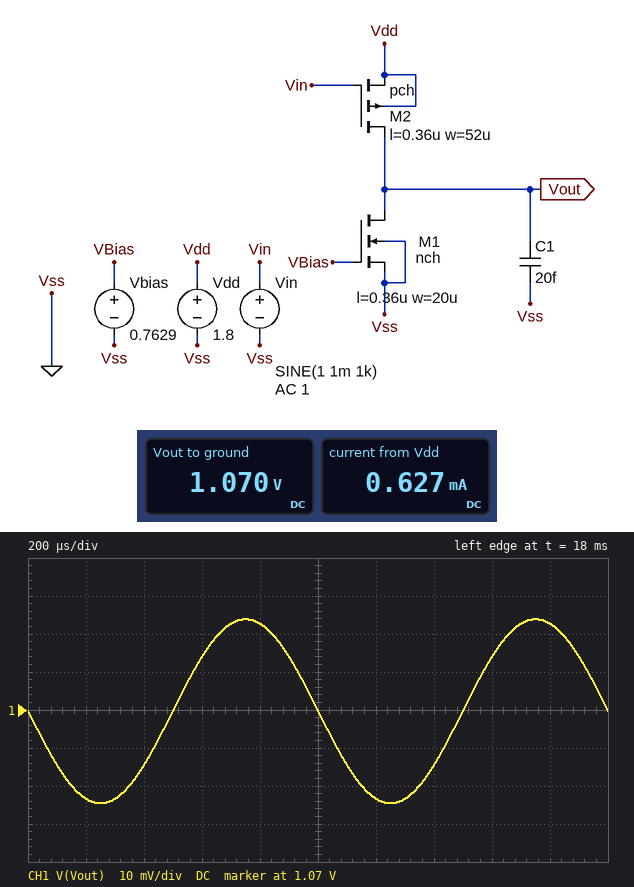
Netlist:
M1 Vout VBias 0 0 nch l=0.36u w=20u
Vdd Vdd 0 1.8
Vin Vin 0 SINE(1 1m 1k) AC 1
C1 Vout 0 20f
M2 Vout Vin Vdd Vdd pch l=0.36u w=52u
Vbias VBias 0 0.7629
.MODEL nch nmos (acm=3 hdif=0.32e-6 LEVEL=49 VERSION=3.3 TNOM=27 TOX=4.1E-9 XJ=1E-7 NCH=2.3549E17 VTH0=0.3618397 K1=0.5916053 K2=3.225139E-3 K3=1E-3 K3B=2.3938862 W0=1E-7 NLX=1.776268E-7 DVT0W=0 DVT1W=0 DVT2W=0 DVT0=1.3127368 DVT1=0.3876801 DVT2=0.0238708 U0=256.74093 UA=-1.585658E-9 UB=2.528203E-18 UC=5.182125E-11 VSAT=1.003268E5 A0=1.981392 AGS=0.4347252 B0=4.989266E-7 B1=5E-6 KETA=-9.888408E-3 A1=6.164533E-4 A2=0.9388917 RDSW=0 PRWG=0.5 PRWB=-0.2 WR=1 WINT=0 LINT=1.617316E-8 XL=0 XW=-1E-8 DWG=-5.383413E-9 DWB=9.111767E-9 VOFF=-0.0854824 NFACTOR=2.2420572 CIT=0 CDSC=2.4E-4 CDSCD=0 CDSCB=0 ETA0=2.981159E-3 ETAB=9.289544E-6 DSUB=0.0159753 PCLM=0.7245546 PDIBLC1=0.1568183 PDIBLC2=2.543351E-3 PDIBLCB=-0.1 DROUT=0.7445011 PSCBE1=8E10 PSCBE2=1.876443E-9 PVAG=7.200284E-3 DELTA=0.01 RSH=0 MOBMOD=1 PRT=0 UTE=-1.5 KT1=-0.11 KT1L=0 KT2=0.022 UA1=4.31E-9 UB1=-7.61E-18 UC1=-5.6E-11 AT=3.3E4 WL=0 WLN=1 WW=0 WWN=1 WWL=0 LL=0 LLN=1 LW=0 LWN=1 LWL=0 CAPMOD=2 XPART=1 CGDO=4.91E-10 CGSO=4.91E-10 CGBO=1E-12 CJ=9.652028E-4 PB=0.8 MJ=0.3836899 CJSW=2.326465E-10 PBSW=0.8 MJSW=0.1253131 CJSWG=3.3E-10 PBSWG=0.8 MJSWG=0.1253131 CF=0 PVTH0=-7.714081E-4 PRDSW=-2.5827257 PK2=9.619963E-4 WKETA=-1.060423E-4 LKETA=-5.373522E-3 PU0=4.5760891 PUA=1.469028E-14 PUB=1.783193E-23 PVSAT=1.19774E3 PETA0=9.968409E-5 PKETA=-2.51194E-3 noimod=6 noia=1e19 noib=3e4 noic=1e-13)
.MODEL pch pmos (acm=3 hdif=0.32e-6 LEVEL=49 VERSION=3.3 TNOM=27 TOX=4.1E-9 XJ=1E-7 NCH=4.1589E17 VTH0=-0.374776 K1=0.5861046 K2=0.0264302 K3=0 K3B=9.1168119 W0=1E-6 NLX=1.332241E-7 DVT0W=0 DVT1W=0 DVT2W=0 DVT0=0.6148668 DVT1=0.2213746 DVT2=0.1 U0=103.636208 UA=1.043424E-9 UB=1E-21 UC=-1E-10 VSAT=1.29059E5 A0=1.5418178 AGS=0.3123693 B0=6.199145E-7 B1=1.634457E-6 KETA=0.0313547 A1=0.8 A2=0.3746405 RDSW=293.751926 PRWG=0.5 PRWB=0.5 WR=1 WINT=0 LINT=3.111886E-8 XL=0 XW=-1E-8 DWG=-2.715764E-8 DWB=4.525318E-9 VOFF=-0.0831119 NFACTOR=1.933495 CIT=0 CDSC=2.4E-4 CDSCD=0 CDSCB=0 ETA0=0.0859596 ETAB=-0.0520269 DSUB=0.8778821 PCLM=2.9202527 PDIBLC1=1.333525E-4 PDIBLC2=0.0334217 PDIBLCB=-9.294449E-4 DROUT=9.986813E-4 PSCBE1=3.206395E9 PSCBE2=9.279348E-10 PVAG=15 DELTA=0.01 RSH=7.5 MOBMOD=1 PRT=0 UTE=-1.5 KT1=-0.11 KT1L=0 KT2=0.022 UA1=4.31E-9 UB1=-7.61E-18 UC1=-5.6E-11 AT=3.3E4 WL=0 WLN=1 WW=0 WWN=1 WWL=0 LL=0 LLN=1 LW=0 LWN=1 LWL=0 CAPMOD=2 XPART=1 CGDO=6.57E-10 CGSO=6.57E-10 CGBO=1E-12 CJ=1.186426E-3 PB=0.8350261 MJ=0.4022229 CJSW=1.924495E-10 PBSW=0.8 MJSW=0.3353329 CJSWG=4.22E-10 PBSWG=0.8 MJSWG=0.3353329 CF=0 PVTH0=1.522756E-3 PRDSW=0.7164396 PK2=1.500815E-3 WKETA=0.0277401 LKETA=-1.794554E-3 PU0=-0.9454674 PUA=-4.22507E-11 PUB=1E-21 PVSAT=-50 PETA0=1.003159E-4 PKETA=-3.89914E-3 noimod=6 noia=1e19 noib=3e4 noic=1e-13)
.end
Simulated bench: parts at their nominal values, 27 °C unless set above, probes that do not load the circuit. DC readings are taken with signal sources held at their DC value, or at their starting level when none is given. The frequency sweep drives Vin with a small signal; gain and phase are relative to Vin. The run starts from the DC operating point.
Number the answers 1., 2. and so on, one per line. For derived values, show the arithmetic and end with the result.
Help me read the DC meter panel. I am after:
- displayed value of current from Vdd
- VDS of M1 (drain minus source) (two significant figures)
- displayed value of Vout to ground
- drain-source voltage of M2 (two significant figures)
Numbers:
1. 0.627 mA
2. 1.07 V = 1.1 V
3. 1.070 V
4. 1.07 V - 1.8 V = -730 mV
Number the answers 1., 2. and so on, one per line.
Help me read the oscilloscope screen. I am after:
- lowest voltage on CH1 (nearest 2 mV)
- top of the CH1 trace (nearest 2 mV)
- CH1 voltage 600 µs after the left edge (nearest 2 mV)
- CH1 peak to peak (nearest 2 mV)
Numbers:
1. 1.046 V
2. 1.094 V
3. 1.084 V
4. 48 mV
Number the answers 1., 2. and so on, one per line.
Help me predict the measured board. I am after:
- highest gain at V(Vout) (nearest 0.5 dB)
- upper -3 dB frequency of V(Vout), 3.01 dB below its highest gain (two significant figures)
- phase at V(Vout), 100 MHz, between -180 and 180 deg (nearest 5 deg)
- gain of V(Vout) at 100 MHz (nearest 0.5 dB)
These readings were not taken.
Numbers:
1. 27.5 dB
2. 150 MHz
3. 145 deg
4. 26.0 dB
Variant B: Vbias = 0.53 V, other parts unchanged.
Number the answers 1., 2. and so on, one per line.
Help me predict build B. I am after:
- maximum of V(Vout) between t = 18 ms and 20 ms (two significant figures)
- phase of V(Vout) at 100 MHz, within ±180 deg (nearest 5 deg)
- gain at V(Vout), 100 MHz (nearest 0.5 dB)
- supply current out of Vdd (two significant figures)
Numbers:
1. 1.8 V
2. 155 deg
3. -27.0 dB
4. 53 µA
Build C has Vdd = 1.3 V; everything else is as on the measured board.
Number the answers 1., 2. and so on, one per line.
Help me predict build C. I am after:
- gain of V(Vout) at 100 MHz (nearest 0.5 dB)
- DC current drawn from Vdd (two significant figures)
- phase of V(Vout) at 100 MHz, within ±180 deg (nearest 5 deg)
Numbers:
1. -46.5 dB
2. 330 nA
3. 110 deg
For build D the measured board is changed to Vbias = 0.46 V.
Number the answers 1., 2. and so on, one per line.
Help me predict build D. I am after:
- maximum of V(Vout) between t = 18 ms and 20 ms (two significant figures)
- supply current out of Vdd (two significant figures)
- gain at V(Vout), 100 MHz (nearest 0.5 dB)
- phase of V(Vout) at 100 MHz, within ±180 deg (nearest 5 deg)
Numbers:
1. 1.8 V
2. 13 µA
3. -34.5 dB
4. 115 deg
